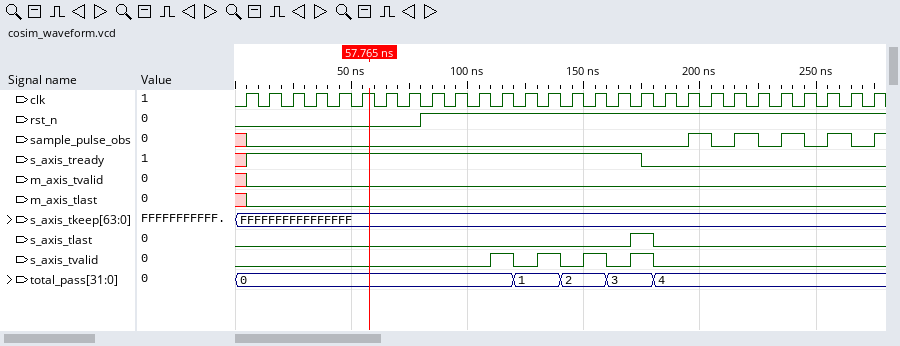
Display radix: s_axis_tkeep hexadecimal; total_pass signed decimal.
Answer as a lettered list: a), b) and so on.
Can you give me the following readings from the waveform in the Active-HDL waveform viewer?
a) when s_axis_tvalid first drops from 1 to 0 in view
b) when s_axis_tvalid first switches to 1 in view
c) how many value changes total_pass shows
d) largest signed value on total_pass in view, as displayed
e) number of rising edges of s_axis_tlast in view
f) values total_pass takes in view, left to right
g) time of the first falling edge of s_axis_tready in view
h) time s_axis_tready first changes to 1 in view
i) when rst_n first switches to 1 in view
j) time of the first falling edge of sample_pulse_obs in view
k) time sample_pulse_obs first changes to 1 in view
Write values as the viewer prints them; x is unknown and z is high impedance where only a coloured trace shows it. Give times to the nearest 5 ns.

a) 120 ns
b) 110 ns
c) 4
d) 4
e) 1
f) 0, 1, 2, 3, 4
g) 175 ns
h) 5 ns
i) 80 ns
j) 205 ns
k) 195 ns
